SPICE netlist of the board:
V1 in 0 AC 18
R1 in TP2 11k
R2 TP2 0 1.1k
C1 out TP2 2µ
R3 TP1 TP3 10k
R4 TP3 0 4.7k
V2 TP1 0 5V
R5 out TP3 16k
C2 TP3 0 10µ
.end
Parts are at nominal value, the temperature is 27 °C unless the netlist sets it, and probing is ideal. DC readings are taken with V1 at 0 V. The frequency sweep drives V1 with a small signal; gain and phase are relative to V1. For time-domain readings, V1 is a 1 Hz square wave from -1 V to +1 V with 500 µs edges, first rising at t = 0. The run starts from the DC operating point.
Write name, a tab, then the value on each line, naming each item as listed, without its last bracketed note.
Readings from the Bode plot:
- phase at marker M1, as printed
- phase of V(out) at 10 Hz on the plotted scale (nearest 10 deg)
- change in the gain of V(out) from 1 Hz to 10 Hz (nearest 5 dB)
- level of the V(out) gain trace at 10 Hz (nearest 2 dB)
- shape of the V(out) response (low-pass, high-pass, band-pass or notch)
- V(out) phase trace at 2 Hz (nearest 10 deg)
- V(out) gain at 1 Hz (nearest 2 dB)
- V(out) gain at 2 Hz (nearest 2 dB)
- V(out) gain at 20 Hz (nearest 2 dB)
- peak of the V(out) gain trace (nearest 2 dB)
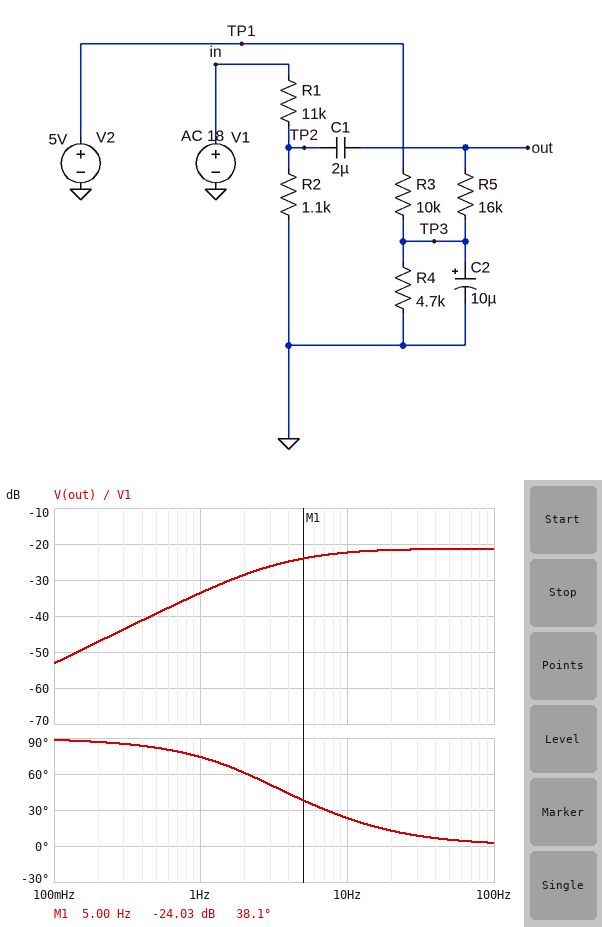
phase at marker M1, as printed	38.1 deg
phase of V(out) at 10 Hz on the plotted scale	20 deg
change in the gain of V(out) from 1 Hz to 10 Hz	10 dB
level of the V(out) gain trace at 10 Hz	-22 dB
shape of the V(out) response	high-pass
V(out) phase trace at 2 Hz	60 deg
V(out) gain at 1 Hz	-34 dB
V(out) gain at 2 Hz	-28 dB
V(out) gain at 20 Hz	-22 dB
peak of the V(out) gain trace	-22 dB
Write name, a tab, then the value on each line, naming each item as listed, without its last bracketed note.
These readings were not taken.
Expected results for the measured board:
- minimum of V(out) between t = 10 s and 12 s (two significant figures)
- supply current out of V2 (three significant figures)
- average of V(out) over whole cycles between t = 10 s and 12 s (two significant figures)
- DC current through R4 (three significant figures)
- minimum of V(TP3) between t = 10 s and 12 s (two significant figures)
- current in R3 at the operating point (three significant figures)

minimum of V(out) between t = 10 s and 12 s	1.4 V
supply current out of V2	340 µA
average of V(out) over whole cycles between t = 10 s and 12 s	1.6 V
DC current through R4	340 µA
minimum of V(TP3) between t = 10 s and 12 s	1.6 V
current in R3 at the operating point	340 µA
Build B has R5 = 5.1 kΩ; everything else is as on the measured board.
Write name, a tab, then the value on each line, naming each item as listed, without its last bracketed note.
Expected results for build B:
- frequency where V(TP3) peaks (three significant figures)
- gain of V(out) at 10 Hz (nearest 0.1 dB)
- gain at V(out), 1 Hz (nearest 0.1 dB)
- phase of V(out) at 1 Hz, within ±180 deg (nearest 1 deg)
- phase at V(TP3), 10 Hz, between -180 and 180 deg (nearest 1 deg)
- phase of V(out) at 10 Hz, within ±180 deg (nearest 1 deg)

frequency where V(TP3) peaks	8.06 Hz
gain of V(out) at 10 Hz	-26.6 dB
gain at V(out), 1 Hz	-40.7 dB
phase of V(out) at 1 Hz, within ±180 deg	79 deg
phase at V(TP3), 10 Hz, between -180 and 180 deg	-10 deg
phase of V(out) at 10 Hz, within ±180 deg	41 deg
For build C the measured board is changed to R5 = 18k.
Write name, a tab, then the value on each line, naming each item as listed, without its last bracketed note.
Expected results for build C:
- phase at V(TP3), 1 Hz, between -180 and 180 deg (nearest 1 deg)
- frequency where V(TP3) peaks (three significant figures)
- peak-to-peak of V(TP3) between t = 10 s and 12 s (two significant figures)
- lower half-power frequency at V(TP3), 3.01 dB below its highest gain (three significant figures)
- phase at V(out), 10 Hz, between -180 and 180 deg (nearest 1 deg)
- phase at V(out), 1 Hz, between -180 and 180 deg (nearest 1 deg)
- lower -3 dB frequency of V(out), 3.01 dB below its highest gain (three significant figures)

phase at V(TP3), 1 Hz, between -180 and 180 deg	63 deg
frequency where V(TP3) peaks	4.57 Hz
peak-to-peak of V(TP3) between t = 10 s and 12 s	23 mV
lower half-power frequency at V(TP3), 3.01 dB below its highest gain	1.77 Hz
phase at V(out), 10 Hz, between -180 and 180 deg	21 deg
phase at V(out), 1 Hz, between -180 and 180 deg	73 deg
lower -3 dB frequency of V(out), 3.01 dB below its highest gain	4.04 Hz
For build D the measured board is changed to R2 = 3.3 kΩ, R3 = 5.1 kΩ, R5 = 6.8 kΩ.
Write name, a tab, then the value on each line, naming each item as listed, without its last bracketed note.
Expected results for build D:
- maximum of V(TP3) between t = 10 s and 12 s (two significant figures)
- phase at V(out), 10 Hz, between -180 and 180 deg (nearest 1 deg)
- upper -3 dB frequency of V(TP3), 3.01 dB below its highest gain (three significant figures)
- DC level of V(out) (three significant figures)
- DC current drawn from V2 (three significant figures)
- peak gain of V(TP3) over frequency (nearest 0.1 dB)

maximum of V(TP3) between t = 10 s and 12 s	2.4 V
phase at V(out), 10 Hz, between -180 and 180 deg	34 deg
upper -3 dB frequency of V(TP3), 3.01 dB below its highest gain	19.6 Hz
DC level of V(out)	2.40 V
DC current drawn from V2	510 µA
peak gain of V(TP3) over frequency	-32.6 dB
